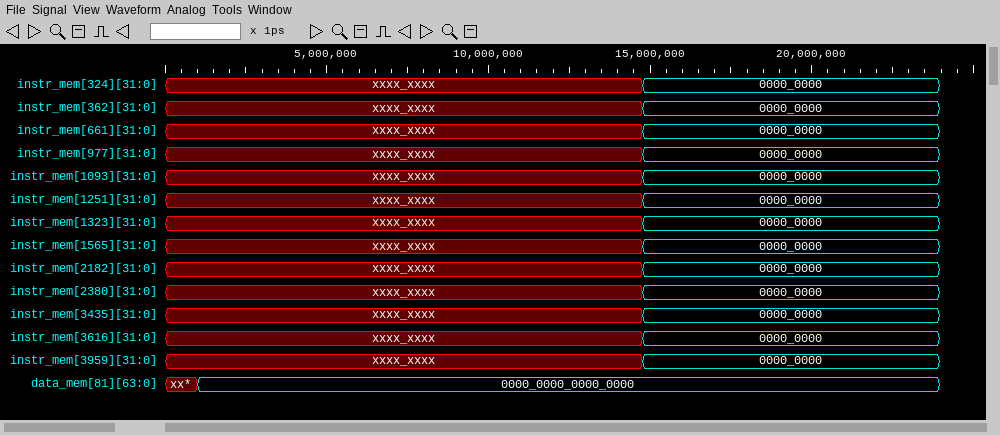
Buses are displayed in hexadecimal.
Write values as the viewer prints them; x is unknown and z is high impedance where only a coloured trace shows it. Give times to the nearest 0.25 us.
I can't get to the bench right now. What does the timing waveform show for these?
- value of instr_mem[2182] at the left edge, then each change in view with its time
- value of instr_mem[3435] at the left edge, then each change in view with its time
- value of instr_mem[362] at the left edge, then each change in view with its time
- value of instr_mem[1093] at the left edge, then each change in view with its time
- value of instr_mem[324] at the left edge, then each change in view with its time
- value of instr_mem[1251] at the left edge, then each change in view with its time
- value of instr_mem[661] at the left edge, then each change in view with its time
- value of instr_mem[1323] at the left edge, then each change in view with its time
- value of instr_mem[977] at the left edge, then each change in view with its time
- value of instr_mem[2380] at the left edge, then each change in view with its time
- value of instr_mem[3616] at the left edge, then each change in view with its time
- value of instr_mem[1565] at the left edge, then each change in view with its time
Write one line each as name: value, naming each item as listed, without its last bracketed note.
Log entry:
value of instr_mem[2182] at the left edge, then each change in view with its time: xxxx_xxxx, 0000_0000 at 14.75 us
value of instr_mem[3435] at the left edge, then each change in view with its time: xxxx_xxxx, 0000_0000 at 14.75 us
value of instr_mem[362] at the left edge, then each change in view with its time: xxxx_xxxx, 0000_0000 at 14.75 us
value of instr_mem[1093] at the left edge, then each change in view with its time: xxxx_xxxx, 0000_0000 at 14.75 us
value of instr_mem[324] at the left edge, then each change in view with its time: xxxx_xxxx, 0000_0000 at 14.75 us
value of instr_mem[1251] at the left edge, then each change in view with its time: xxxx_xxxx, 0000_0000 at 14.75 us
value of instr_mem[661] at the left edge, then each change in view with its time: xxxx_xxxx, 0000_0000 at 14.75 us
value of instr_mem[1323] at the left edge, then each change in view with its time: xxxx_xxxx, 0000_0000 at 14.75 us
value of instr_mem[977] at the left edge, then each change in view with its time: xxxx_xxxx, 0000_0000 at 14.75 us
value of instr_mem[2380] at the left edge, then each change in view with its time: xxxx_xxxx, 0000_0000 at 14.75 us
value of instr_mem[3616] at the left edge, then each change in view with its time: xxxx_xxxx, 0000_0000 at 14.75 us
value of instr_mem[1565] at the left edge, then each change in view with its time: xxxx_xxxx, 0000_0000 at 14.75 us
